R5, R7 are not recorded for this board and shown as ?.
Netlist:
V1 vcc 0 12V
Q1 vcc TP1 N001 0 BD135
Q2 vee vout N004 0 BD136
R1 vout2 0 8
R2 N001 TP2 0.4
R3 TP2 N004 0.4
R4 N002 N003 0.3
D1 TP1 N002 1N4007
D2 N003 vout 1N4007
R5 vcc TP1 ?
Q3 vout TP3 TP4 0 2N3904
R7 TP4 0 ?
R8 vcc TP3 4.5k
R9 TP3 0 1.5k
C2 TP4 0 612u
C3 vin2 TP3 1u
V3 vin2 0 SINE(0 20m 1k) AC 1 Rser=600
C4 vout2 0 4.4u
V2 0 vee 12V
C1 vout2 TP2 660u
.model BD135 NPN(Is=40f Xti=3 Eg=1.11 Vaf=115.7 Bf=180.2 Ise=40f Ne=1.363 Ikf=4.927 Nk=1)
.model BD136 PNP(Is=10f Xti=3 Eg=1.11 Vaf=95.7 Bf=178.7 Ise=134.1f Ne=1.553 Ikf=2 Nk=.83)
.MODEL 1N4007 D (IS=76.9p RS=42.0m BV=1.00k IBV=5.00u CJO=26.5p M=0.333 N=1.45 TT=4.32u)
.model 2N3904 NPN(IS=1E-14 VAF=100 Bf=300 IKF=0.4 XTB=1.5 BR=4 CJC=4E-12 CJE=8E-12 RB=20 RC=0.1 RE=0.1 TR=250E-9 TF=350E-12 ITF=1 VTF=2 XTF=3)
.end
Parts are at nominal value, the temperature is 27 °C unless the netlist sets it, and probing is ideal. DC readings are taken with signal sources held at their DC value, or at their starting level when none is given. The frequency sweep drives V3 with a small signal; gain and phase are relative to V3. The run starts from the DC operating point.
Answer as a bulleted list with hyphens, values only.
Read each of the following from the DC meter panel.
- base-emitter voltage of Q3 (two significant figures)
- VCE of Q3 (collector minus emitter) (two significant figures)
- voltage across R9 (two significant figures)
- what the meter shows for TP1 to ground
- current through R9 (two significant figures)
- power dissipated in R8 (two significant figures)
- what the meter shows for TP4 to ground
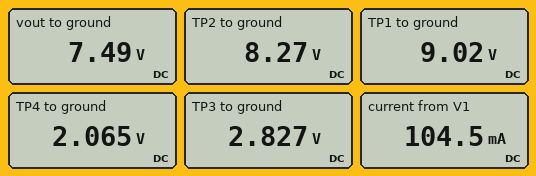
- 760 mV
- 5.4 V
- 2.8 V
- 9.02 V
- 1.9 mA
- 19 mW
- 2.065 V
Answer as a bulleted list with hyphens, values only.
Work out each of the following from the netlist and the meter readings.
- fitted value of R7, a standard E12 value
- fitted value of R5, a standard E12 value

- 47 Ω
- 68 Ω
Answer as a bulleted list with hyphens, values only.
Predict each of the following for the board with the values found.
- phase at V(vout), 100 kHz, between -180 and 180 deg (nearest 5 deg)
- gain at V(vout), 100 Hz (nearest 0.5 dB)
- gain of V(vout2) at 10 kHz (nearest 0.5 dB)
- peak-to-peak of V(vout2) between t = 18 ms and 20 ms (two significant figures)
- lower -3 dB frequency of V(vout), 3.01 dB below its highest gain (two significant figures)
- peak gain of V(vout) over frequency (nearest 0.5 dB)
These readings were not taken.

- 160 deg
- 15.0 dB
- 24.5 dB
- 650 mV
- 280 Hz
- 25.0 dB
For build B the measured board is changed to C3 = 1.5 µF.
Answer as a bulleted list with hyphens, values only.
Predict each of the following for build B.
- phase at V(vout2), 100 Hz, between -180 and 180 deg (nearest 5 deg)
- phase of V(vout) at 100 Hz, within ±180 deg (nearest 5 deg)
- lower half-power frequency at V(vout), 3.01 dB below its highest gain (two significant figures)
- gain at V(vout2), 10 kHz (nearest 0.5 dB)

- -85 deg
- -100 deg
- 220 Hz
- 24.5 dB
